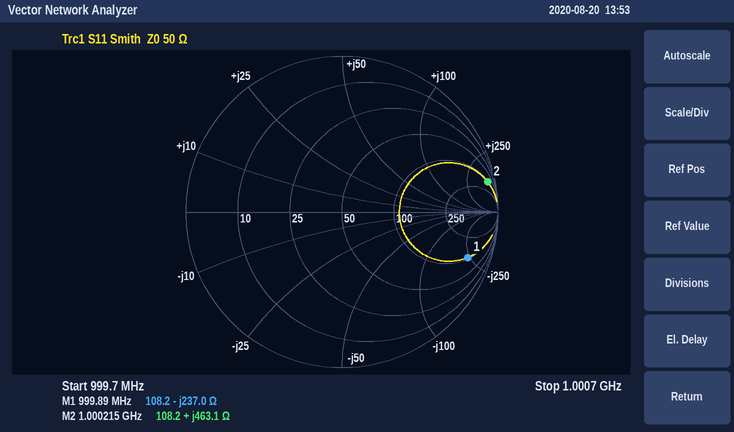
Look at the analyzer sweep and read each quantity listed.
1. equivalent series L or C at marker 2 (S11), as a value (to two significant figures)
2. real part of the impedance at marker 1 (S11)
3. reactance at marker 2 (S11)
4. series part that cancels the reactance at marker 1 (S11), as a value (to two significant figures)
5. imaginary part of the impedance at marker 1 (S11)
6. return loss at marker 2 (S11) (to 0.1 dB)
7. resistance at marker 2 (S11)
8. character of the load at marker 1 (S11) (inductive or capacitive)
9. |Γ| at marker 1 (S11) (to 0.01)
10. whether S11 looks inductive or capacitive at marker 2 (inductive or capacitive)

74 nH
108.2 Ω
+463.1 Ω
38 nH
-237.0 Ω
0.4 dB
108.2 Ω
capacitive
0.86
inductive
